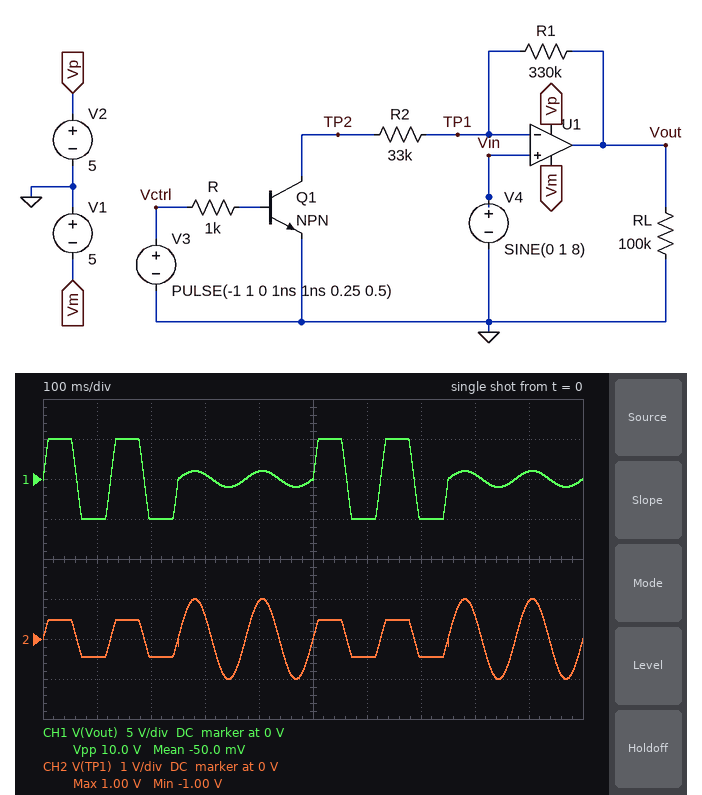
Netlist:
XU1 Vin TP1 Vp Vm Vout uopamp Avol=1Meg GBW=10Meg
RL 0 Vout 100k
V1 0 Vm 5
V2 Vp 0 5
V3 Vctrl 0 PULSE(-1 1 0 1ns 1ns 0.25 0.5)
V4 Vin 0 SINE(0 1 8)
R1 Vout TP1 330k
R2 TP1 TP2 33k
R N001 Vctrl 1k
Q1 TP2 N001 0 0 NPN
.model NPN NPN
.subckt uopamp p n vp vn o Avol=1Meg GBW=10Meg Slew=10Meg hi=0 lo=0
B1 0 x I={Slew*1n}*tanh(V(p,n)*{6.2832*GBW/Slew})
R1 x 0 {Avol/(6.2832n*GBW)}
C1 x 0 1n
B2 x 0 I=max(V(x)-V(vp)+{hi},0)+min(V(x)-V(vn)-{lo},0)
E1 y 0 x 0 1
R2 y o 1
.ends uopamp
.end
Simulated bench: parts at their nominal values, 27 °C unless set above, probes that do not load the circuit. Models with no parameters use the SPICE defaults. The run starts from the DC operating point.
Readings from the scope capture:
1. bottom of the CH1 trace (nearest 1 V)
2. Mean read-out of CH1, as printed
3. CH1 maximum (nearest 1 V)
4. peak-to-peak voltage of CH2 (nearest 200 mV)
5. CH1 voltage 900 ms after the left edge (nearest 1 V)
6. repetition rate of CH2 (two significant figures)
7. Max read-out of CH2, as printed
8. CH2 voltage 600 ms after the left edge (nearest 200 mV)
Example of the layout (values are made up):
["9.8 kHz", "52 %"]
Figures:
["-5 V", "-50.0 mV", "5 V", "2.0 V", "1 V", "8.0 Hz", "1.00 V", "-400 mV"]
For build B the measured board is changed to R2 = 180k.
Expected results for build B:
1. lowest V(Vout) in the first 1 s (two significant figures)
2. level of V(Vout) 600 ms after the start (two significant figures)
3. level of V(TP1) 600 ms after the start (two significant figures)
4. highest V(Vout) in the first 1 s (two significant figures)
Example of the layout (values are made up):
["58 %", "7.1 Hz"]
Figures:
["-2.9 V", "-2.7 V", "-950 mV", "2.8 V"]
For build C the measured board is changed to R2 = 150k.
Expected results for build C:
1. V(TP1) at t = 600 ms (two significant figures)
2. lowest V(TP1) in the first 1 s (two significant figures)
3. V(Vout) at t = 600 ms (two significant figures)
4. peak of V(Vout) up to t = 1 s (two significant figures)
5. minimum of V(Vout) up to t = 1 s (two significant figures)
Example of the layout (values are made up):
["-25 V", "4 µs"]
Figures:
["-950 mV", "-1.0 V", "-3.1 V", "3.2 V", "-3.2 V"]
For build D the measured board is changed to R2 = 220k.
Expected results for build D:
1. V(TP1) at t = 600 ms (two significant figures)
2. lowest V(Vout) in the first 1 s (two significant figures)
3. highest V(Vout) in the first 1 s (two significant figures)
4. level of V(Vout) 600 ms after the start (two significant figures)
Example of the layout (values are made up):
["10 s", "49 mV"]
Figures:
["-950 mV", "-2.5 V", "2.5 V", "-2.4 V"]
